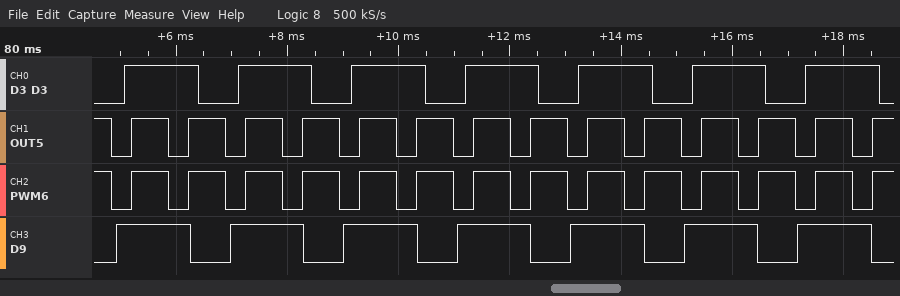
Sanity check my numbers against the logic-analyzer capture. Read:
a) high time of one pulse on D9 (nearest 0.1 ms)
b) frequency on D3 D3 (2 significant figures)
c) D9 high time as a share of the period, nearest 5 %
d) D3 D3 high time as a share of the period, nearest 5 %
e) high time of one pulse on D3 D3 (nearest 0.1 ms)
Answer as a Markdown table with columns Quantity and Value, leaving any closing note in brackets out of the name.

| Quantity | Value |
|---|---|
| high time of one pulse on D9 | 1.3 ms |
| frequency on D3 D3 | 490 Hz |
| D9 high time as a share of the period, nearest 5 % | 65 % |
| D3 D3 high time as a share of the period, nearest 5 % | 65 % |
| high time of one pulse on D3 D3 | 1.3 ms |
